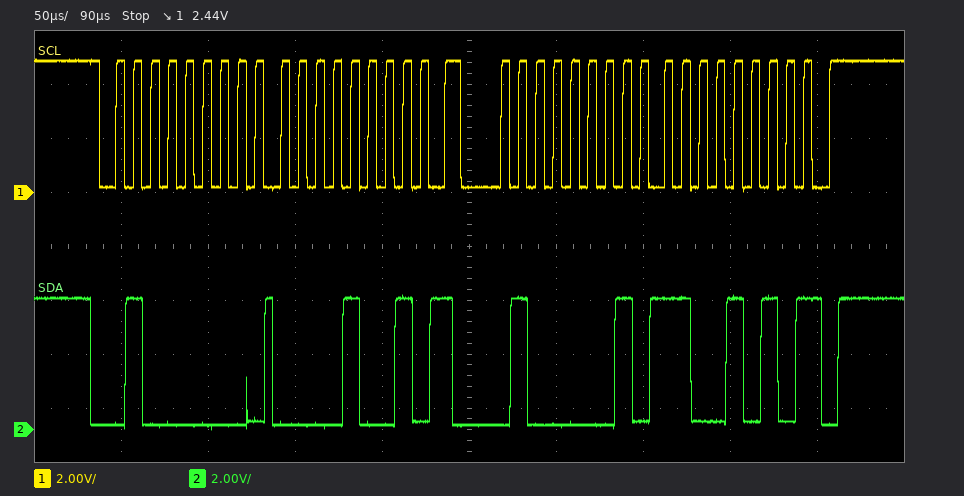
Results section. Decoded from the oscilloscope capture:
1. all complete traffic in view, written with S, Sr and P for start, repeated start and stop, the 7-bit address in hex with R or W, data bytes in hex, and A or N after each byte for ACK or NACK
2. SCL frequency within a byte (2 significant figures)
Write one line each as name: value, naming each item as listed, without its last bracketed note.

all complete traffic in view, written with S, Sr and P for start, repeated start and stop, the 7-bit address in hex with R or W, data bytes in hex, and A or N after each byte for ACK or NACK: S 20W A 09 A Sr 20R A CA N P
SCL frequency within a byte: 100 kHz
